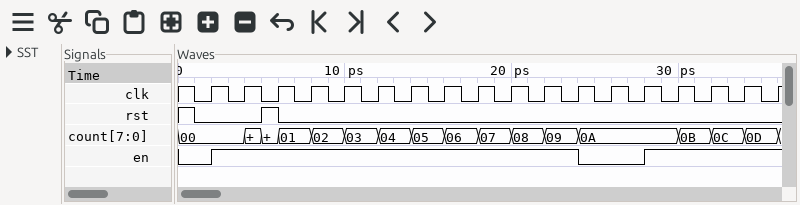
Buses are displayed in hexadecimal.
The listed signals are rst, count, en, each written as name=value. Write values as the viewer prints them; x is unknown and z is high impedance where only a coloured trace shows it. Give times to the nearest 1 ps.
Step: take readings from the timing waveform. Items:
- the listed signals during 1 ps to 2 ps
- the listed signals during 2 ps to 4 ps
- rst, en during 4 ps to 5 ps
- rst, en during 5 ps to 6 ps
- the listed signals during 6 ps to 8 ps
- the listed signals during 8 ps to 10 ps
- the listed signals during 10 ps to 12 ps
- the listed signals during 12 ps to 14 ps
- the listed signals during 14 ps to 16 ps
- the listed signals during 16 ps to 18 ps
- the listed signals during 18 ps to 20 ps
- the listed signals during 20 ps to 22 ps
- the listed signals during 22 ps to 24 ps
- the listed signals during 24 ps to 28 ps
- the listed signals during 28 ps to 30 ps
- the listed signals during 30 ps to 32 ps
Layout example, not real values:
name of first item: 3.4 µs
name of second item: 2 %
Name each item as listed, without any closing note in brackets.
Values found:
the listed signals during 1 ps to 2 ps: rst=0, count=00, en=0
the listed signals during 2 ps to 4 ps: rst=0, count=00, en=1
rst, en during 4 ps to 5 ps: rst=0, en=1
rst, en during 5 ps to 6 ps: rst=1, en=1
the listed signals during 6 ps to 8 ps: rst=0, count=01, en=1
the listed signals during 8 ps to 10 ps: rst=0, count=02, en=1
the listed signals during 10 ps to 12 ps: rst=0, count=03, en=1
the listed signals during 12 ps to 14 ps: rst=0, count=04, en=1
the listed signals during 14 ps to 16 ps: rst=0, count=05, en=1
the listed signals during 16 ps to 18 ps: rst=0, count=06, en=1
the listed signals during 18 ps to 20 ps: rst=0, count=07, en=1
the listed signals during 20 ps to 22 ps: rst=0, count=08, en=1
the listed signals during 22 ps to 24 ps: rst=0, count=09, en=1
the listed signals during 24 ps to 28 ps: rst=0, count=0A, en=0
the listed signals during 28 ps to 30 ps: rst=0, count=0A, en=1
the listed signals during 30 ps to 32 ps: rst=0, count=0B, en=1
